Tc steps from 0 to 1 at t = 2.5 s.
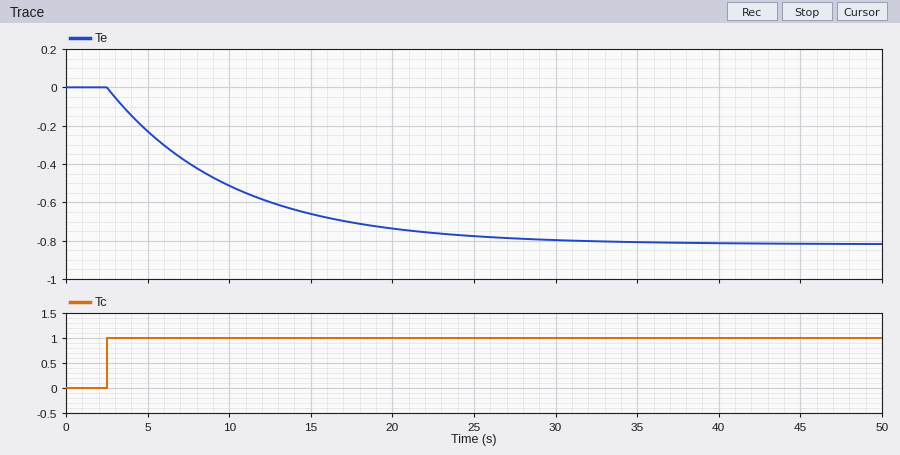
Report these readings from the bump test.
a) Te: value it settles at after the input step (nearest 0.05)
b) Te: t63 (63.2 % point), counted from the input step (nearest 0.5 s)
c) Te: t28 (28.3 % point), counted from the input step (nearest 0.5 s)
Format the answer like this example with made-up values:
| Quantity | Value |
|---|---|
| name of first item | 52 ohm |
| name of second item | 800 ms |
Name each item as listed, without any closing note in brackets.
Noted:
| Quantity | Value |
|---|---|
| Te: value it settles at after the input step | -0.80 |
| Te: t63 (63.2 % point), counted from the input step | 7.5 s |
| Te: t28 (28.3 % point), counted from the input step | 2.5 s |
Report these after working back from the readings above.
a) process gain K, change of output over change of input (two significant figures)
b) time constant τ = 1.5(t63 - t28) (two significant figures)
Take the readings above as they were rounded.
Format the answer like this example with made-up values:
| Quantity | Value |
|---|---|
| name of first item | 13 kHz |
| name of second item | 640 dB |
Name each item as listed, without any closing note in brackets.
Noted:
| Quantity | Value |
|---|---|
| process gain K, change of output over change of input | -0.80 |
| time constant τ = 1.5(t63 - t28) | 7.5 s |
